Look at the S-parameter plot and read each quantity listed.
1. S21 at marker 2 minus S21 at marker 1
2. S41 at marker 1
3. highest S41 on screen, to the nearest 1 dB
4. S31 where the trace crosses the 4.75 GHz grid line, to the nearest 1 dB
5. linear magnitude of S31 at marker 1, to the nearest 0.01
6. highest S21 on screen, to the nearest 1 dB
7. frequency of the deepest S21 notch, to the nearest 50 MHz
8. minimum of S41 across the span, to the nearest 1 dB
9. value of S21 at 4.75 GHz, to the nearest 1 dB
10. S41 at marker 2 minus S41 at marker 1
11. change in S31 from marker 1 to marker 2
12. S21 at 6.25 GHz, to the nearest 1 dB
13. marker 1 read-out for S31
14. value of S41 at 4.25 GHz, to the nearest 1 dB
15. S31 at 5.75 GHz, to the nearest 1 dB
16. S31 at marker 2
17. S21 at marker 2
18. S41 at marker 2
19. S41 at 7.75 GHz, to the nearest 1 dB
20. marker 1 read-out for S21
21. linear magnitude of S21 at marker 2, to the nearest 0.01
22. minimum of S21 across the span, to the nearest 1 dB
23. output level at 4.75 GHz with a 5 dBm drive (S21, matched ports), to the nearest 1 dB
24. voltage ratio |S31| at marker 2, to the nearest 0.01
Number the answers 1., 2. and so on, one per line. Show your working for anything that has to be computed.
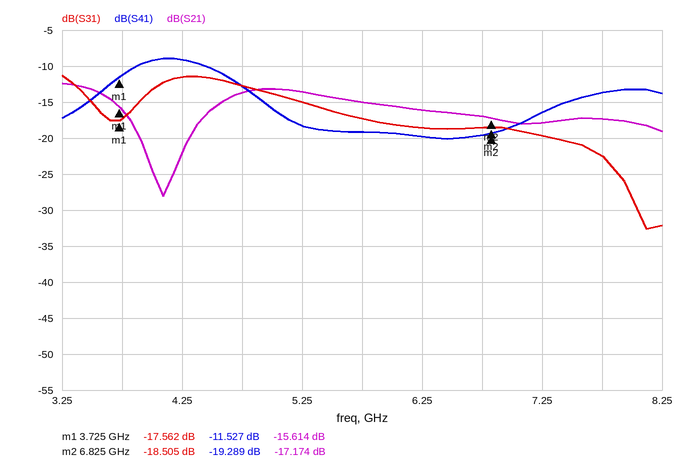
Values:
1. -17.174 − (-15.614) = -1.560 dB
2. -11.527 dB
3. -9 dB
4. -13 dB
5. 10^(-17.562/20) ≈ 0.13
6. -12 dB
7. 4.10 GHz
8. -20 dB
9. -14 dB
10. -19.289 − (-11.527) = -7.762 dB
11. -18.505 − (-17.562) = -0.943 dB
12. -16 dB
13. -17.562 dB
14. -9 dB
15. -17 dB
16. -18.505 dB
17. -17.174 dB
18. -19.289 dB
19. -14 dB
20. -15.614 dB
21. 10^(-17.174/20) ≈ 0.14
22. -28 dB
23. 5 dBm + (-14 dB) = -9 dBm
24. 10^(-18.505/20) ≈ 0.12
